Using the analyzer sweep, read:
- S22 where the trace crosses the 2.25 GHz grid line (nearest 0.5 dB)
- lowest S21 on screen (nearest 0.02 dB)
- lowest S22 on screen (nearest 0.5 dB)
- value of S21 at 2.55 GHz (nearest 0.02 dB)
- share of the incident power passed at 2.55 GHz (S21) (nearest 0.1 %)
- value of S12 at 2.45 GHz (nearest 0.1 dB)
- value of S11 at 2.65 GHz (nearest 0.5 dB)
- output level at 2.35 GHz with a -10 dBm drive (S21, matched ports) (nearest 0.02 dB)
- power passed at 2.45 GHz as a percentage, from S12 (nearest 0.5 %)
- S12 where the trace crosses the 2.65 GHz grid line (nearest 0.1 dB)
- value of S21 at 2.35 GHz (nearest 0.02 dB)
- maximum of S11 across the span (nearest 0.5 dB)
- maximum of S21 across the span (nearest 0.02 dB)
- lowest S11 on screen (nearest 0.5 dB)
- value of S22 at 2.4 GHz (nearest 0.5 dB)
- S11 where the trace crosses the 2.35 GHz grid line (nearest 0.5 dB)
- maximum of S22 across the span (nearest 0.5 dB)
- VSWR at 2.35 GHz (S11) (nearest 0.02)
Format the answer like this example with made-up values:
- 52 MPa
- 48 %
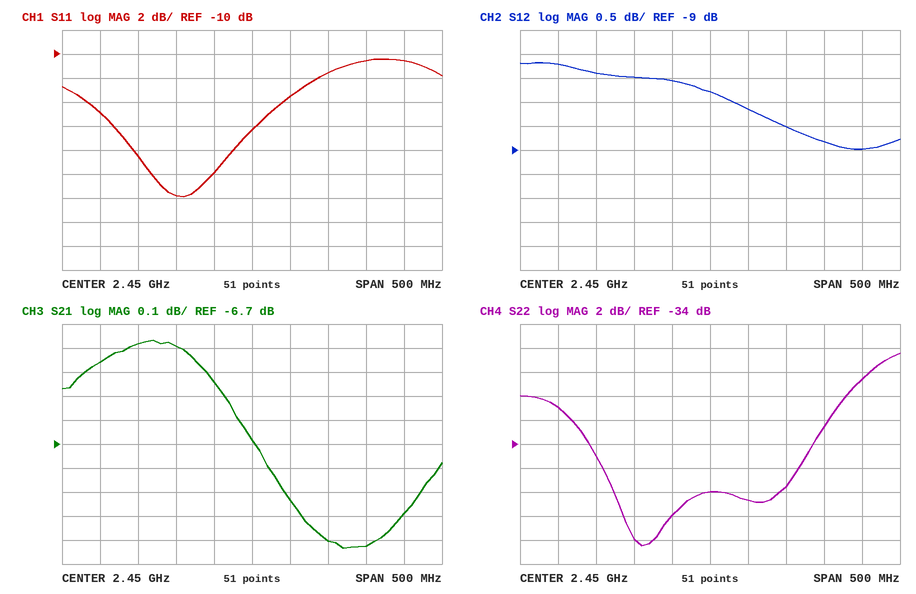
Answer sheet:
- -31.0 dB
- -7.14 dB
- -42.5 dB
- -7.10 dB
- 19.5 %
- -7.8 dB
- -10.5 dB
- -16.30 dBm
- 16.5 %
- -9.0 dB
- -6.30 dB
- -10.5 dB
- -6.26 dB
- -22.0 dB
- -40.0 dB
- -22.0 dB
- -26.5 dB
- 1.18
